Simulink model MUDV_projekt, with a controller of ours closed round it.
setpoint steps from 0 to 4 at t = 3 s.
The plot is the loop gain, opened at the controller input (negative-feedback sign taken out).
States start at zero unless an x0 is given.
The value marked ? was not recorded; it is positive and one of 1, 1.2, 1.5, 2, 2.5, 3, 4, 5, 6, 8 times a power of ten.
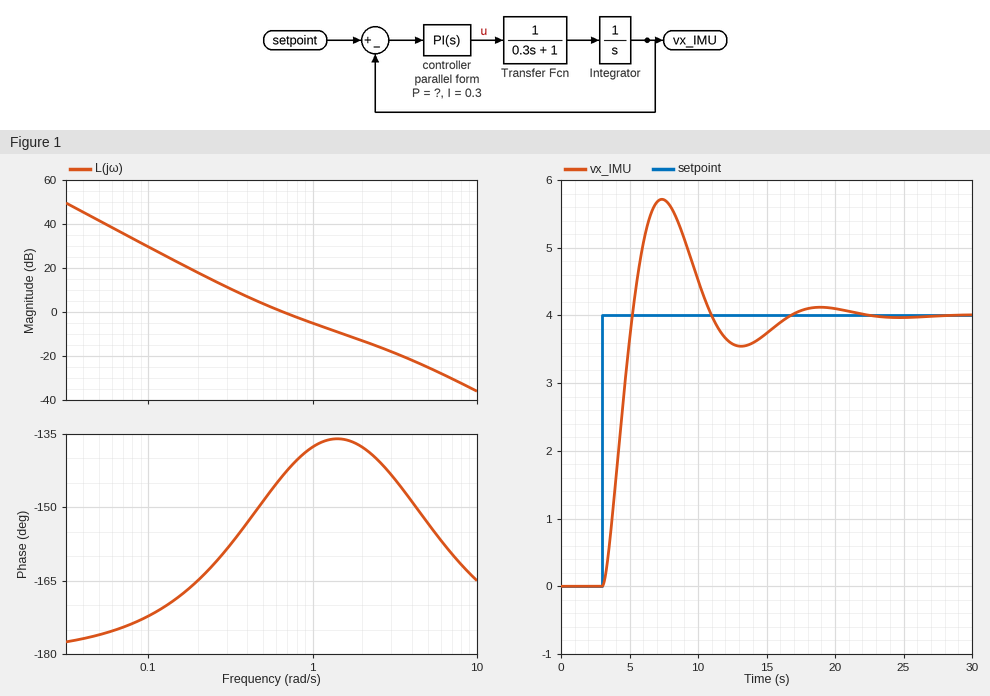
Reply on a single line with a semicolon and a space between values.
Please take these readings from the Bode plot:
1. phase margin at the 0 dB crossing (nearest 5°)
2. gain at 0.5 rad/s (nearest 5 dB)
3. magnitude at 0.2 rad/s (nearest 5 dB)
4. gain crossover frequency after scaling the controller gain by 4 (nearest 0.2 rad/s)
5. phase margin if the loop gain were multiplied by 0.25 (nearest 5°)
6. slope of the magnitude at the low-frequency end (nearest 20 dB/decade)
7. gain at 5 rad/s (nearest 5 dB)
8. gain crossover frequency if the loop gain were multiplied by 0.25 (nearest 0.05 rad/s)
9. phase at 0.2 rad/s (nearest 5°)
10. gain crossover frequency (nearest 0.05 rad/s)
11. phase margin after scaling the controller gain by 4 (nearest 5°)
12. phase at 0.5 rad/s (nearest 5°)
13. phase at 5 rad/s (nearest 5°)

35°; 5 dB; 20 dB; 1.8 rad/s; 20°; -40 dB/decade; -25 dB; 0.30 rad/s; -165°; 0.65 rad/s; 45°; -150°; -155°
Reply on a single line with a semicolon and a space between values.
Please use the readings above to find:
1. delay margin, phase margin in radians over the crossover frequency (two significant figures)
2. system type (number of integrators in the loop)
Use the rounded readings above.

0.94 s; 2
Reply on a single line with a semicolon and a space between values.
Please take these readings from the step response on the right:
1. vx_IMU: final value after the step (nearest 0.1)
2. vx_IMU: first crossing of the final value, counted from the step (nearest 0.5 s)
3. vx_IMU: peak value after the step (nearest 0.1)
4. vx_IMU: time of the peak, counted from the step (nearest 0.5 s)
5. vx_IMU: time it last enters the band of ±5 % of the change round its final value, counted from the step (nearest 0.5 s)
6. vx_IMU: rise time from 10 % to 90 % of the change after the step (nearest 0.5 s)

4.0; 2.0 s; 5.7; 4.5 s; 12.5 s; 1.5 s
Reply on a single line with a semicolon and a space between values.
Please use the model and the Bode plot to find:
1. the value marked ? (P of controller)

0.5
